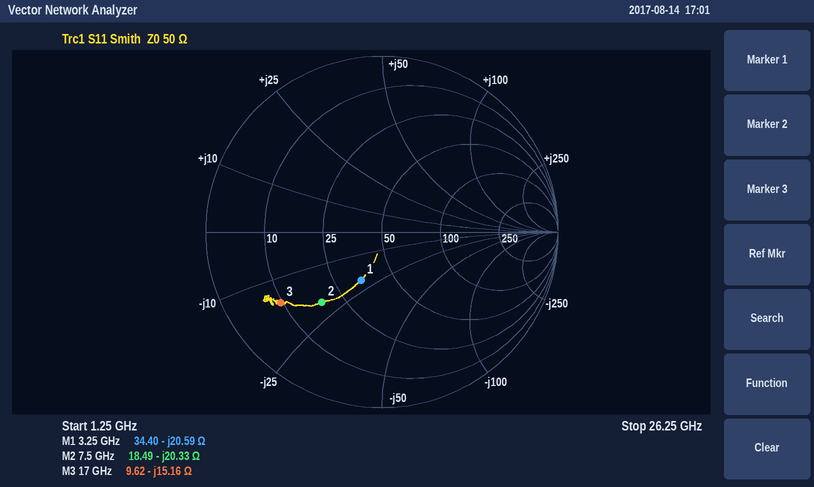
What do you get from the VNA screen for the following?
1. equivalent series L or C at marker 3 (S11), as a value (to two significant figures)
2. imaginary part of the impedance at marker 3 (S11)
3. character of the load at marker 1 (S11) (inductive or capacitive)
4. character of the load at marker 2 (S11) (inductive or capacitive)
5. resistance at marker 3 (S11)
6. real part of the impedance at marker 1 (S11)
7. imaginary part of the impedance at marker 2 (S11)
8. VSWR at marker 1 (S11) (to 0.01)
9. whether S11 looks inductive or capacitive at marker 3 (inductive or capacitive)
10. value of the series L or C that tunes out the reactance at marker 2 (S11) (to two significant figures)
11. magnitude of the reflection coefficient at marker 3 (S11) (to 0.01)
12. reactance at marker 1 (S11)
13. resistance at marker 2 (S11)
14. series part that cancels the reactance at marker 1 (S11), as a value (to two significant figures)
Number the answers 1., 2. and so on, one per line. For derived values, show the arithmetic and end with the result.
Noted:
1. C = 1/(2π × 17 GHz × 15.16 Ω) ≈ 618 fF, so 620 fF to two significant figures
2. -15.16 Ω
3. capacitive
4. capacitive
5. 9.62 Ω
6. 34.40 Ω
7. -20.33 Ω
8. 1.85
9. capacitive
10. L = 20.33 Ω/(2π × 7.5 GHz) ≈ 431 pH, so 430 pH to two significant figures
11. 0.70
12. -20.59 Ω
13. 18.49 Ω
14. L = 20.59 Ω/(2π × 3.25 GHz) ≈ 1.0 nH
